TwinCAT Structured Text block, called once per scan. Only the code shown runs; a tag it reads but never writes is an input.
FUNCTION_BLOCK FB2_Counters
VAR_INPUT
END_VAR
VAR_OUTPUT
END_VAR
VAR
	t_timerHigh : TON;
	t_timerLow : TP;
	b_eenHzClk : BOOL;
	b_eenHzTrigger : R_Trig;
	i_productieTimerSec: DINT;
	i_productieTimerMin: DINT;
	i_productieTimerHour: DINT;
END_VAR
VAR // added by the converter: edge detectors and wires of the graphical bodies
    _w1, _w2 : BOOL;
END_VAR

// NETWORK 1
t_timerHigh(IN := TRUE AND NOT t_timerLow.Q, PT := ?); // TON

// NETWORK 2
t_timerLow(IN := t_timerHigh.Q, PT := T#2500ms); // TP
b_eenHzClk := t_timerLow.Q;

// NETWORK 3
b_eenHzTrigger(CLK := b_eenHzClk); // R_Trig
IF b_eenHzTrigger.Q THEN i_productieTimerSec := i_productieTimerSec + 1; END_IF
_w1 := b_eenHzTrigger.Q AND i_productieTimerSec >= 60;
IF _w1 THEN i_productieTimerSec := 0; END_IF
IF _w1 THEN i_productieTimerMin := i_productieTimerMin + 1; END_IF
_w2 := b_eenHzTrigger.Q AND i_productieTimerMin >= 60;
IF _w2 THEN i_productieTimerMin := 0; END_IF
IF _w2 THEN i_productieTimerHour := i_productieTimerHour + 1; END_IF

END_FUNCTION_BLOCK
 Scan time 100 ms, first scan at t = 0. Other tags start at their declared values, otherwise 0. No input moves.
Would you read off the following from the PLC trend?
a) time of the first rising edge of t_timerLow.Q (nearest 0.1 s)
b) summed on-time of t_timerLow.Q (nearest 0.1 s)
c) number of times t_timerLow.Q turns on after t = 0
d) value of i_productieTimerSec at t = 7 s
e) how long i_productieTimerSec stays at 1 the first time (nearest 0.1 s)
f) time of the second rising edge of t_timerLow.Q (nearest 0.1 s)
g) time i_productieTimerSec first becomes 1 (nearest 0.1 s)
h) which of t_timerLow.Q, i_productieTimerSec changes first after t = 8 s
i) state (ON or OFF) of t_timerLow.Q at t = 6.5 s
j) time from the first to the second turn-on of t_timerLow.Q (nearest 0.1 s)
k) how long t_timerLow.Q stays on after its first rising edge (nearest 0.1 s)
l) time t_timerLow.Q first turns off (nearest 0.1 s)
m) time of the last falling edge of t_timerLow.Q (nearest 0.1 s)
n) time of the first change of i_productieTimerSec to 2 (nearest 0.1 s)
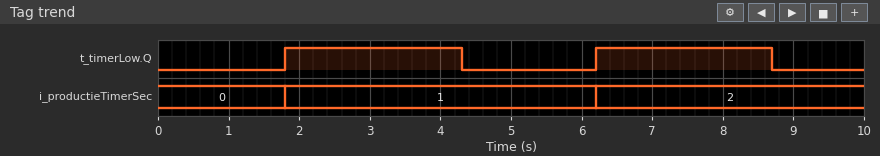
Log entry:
1.8 s
5.0 s
2
2
4.4 s
6.2 s
1.8 s
t_timerLow.Q
ON
4.4 s
2.5 s
4.3 s
8.7 s
6.2 s
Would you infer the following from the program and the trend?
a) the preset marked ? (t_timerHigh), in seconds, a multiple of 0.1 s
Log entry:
1.8 s
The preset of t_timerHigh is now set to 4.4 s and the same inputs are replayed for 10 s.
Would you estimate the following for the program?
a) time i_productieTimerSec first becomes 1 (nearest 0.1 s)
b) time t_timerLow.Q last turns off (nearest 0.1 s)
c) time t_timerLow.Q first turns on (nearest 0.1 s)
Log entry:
4.4 s
6.9 s
4.4 s
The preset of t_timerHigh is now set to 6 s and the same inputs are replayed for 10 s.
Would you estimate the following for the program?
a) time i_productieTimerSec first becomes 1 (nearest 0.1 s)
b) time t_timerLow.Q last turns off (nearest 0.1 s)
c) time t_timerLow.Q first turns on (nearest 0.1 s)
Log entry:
6.0 s
8.5 s
6.0 s
